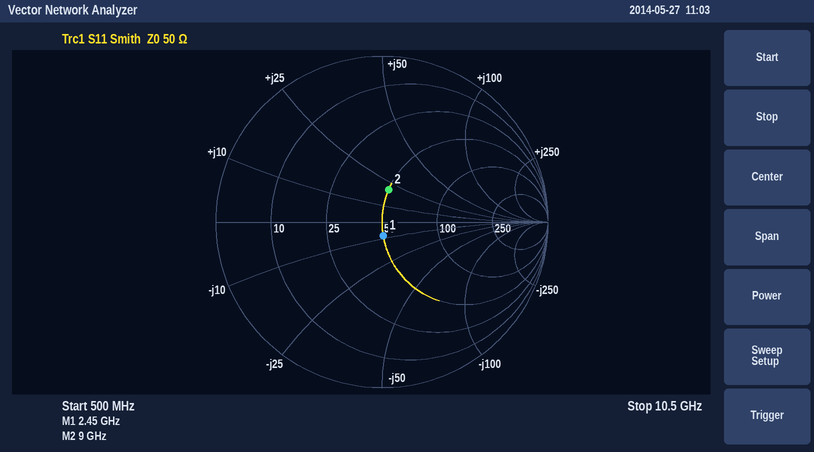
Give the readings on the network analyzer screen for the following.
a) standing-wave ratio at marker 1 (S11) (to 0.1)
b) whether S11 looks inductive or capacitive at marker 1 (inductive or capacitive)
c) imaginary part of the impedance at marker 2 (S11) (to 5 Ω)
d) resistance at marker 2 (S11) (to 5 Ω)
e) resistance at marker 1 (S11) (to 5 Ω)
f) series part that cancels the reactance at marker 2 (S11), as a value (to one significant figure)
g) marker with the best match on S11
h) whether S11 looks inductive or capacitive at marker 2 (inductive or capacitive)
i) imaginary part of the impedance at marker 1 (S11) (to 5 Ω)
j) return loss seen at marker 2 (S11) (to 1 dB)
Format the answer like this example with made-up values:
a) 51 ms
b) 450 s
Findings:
a) 1.2
b) capacitive
c) +20 Ω
d) 50 Ω
e) 50 Ω
f) 900 fF
g) marker 1
h) inductive
i) -10 Ω
j) 14 dB
